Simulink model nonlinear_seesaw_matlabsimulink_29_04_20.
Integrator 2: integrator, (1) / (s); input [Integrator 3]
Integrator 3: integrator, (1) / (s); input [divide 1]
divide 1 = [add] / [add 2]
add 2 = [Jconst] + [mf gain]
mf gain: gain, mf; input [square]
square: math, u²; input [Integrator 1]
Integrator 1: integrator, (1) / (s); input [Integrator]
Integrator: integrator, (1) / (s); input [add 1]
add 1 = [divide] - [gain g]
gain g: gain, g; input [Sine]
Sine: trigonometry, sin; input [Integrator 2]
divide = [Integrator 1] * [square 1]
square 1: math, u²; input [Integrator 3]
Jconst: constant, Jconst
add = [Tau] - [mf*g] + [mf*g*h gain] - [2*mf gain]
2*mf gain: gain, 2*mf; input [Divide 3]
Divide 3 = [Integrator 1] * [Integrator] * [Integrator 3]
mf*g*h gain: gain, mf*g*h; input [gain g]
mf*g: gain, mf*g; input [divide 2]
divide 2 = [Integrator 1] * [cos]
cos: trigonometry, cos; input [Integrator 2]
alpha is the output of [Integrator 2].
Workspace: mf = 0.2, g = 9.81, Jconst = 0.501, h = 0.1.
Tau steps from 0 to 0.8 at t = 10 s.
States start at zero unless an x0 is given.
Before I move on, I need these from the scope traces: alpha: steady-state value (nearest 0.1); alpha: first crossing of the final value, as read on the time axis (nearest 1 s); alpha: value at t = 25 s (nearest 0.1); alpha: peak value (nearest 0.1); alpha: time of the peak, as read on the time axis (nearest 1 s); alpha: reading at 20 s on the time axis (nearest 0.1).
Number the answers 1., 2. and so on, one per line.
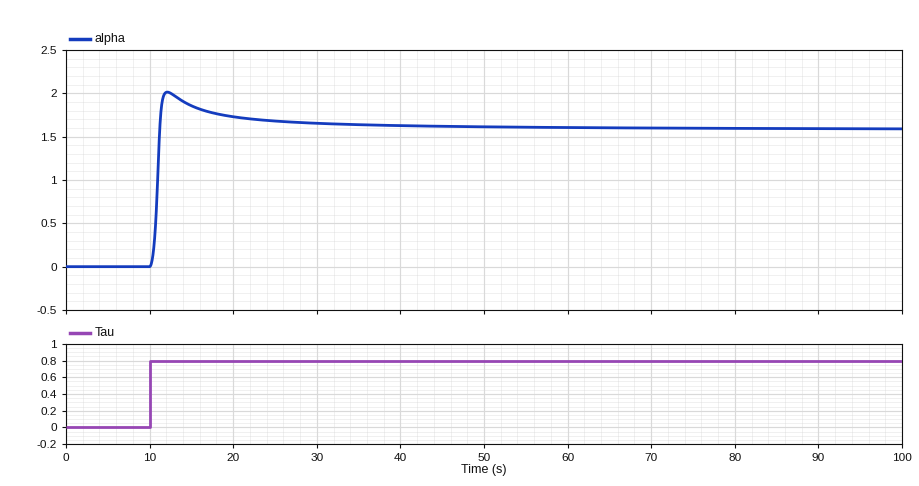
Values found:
1. 1.6
2. 11 s
3. 1.7
4. 2.0
5. 12 s
6. 1.7
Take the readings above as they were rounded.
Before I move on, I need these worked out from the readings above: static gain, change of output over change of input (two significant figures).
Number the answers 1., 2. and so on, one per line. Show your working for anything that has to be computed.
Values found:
1. (1.6 - 0) / (0.8 - 0) = 2.0
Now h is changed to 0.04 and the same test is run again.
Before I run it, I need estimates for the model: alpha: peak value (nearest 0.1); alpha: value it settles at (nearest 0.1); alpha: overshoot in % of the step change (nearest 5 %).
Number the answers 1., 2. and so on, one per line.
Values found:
1. 1.8
2. 1.6
3. 15 %
